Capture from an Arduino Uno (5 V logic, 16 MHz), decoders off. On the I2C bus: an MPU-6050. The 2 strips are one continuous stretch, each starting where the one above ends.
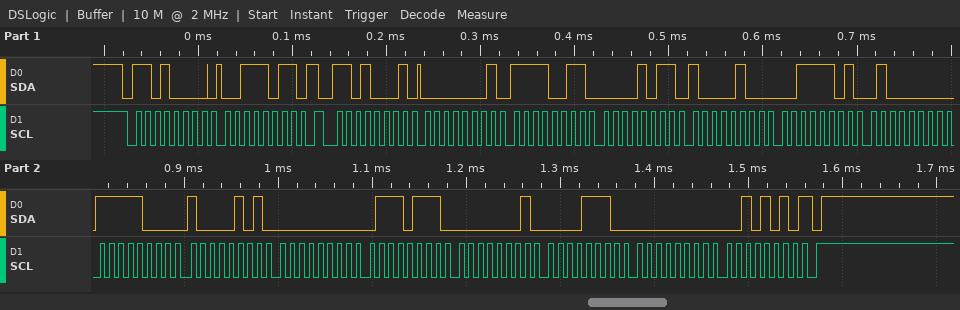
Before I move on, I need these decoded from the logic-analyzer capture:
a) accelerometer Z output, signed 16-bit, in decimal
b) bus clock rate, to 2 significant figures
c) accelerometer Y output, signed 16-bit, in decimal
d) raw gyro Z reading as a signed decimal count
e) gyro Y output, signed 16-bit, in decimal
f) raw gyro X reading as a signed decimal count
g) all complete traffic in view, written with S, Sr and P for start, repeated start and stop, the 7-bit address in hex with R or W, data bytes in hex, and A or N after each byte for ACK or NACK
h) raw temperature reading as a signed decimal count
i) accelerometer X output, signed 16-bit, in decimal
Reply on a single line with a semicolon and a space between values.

15680; 100 kHz; 2948; 42; 270; 119; S 68W A 3B A Sr 68R A 01 A F3 A 0B A 84 A 3D A 40 A F8 A 85 A 00 A 77 A 01 A 0E A 00 A 2A N P; -1915; 499
